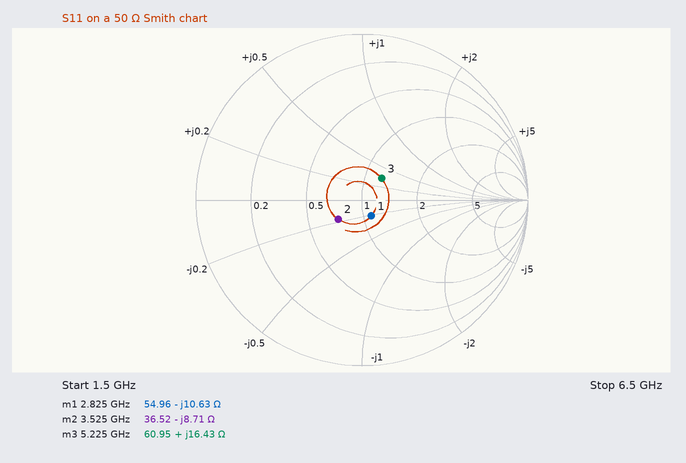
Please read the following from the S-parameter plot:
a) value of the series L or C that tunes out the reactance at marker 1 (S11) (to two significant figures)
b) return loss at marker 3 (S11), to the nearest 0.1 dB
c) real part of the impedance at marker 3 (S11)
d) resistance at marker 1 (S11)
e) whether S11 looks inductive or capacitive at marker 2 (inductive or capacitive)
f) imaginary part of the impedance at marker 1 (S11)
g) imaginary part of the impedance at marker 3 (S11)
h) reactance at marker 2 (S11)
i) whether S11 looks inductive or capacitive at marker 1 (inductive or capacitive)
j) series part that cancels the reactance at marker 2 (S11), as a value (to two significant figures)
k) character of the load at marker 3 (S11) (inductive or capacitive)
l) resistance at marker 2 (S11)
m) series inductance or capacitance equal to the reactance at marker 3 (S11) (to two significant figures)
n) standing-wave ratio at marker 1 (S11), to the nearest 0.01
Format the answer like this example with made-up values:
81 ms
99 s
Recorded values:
600 pH
15.1 dB
60.95 Ω
54.96 Ω
capacitive
-10.63 Ω
+16.43 Ω
-8.71 Ω
capacitive
390 pH
inductive
36.52 Ω
500 pH
1.25
